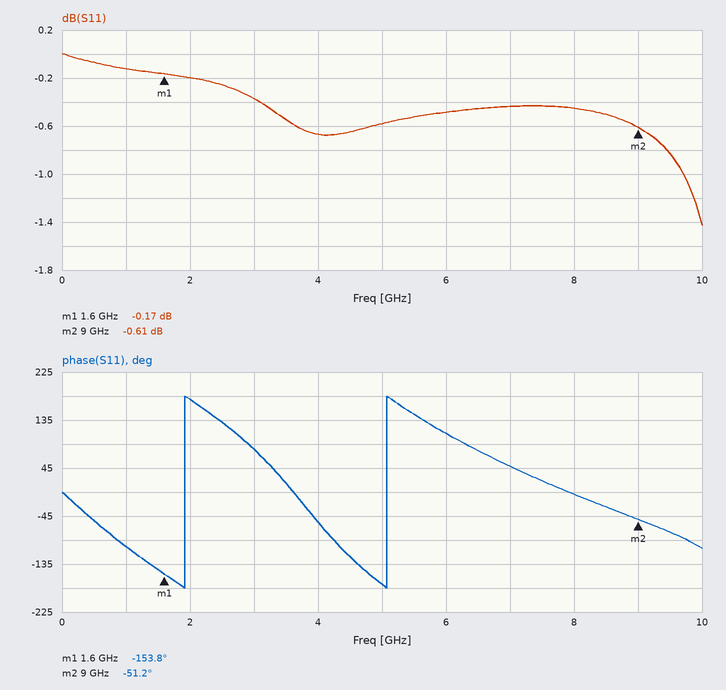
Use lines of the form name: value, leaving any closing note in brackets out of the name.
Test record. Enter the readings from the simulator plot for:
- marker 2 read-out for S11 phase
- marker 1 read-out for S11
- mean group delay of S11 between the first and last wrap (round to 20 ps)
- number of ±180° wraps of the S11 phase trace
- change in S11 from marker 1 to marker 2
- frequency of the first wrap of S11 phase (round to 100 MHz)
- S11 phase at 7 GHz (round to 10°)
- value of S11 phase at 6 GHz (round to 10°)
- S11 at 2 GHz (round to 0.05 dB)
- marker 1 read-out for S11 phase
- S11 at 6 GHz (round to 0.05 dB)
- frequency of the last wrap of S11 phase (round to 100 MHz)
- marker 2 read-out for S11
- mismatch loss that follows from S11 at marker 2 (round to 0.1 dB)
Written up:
marker 2 read-out for S11 phase: -51.2°
marker 1 read-out for S11: -0.17 dB
mean group delay of S11 between the first and last wrap: 320 ps
number of ±180° wraps of the S11 phase trace: 2
change in S11 from marker 1 to marker 2: -0.44 dB
frequency of the first wrap of S11 phase: 1.9 GHz
S11 phase at 7 GHz: 50°
value of S11 phase at 6 GHz: 110°
S11 at 2 GHz: -0.20 dB
marker 1 read-out for S11 phase: -153.8°
S11 at 6 GHz: -0.50 dB
frequency of the last wrap of S11 phase: 5.1 GHz
marker 2 read-out for S11: -0.61 dB
mismatch loss that follows from S11 at marker 2: 8.8 dB
